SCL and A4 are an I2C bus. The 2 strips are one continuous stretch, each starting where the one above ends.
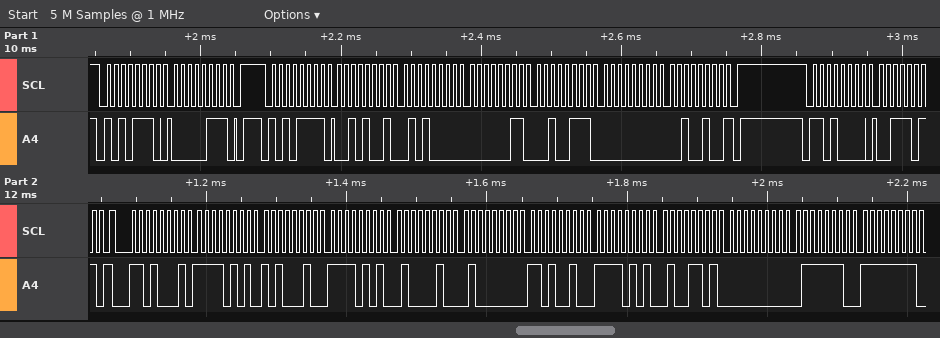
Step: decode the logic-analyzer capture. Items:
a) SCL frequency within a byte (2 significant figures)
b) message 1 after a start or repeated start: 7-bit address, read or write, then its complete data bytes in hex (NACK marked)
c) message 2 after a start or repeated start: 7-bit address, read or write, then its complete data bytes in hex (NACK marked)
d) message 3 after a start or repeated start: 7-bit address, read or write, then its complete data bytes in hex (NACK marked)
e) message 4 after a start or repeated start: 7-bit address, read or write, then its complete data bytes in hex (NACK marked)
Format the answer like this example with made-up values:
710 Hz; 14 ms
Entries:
100 kHz; 0x57 write: 07; 0x57 read: 29 50 03 27 00 24 NACK; 0x68 write: 3B; 0x68 read: F5 A2 F5 42 40 D2 F5 4D 00 7E FF
